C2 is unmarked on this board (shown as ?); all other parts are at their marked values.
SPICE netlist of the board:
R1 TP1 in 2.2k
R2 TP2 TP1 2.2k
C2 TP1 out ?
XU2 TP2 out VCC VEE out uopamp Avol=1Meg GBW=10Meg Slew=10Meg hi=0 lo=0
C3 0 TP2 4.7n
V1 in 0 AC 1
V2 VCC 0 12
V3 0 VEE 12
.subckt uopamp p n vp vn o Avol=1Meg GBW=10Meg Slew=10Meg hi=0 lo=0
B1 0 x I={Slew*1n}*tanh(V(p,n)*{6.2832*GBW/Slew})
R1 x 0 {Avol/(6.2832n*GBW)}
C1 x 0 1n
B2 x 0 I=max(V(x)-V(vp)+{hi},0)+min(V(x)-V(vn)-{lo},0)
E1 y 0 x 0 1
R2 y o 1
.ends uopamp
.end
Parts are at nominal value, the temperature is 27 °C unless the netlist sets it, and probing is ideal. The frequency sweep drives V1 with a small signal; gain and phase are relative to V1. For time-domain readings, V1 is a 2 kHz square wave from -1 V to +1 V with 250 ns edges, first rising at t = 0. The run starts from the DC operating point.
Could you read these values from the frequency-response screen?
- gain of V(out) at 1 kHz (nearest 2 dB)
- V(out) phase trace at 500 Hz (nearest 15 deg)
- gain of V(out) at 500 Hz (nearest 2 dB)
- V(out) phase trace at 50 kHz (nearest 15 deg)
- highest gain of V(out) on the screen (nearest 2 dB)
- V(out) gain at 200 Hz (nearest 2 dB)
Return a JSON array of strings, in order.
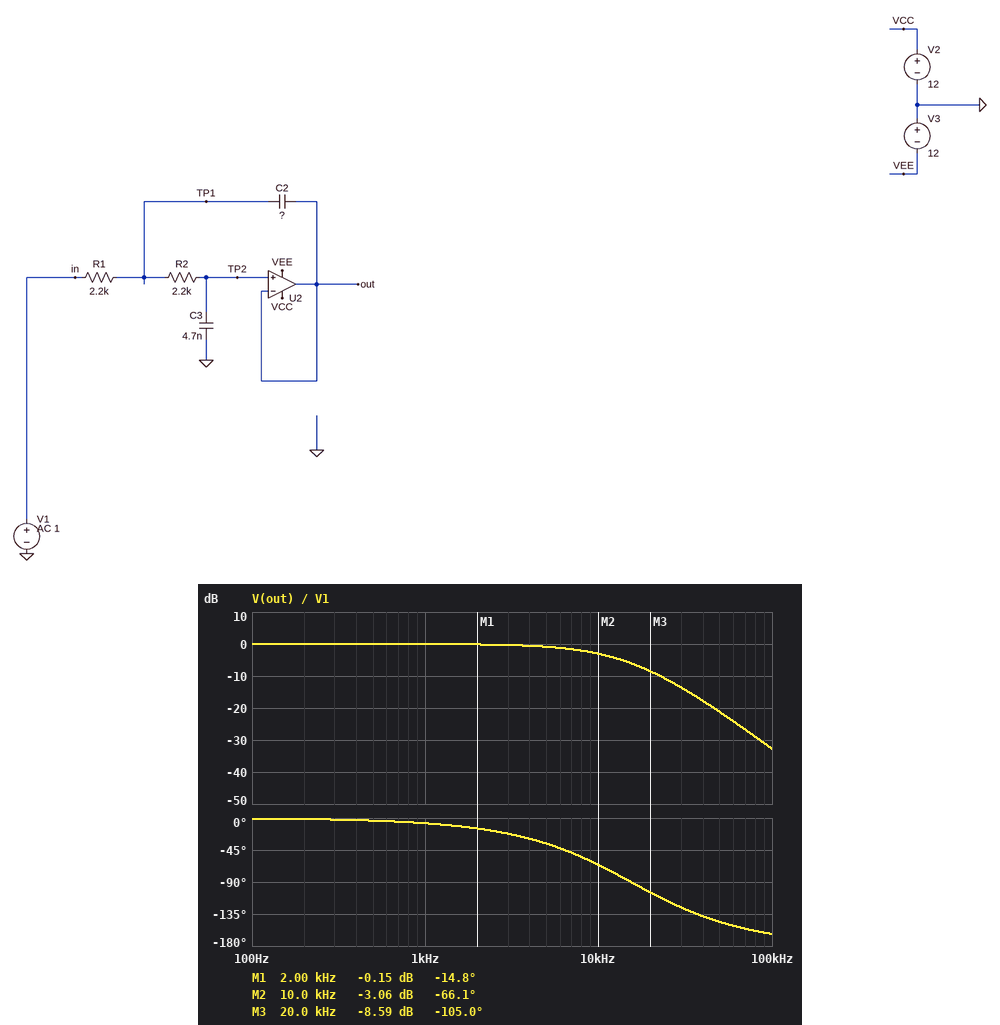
["0 dB", "0 deg", "0 dB", "-150 deg", "0 dB", "0 dB"]
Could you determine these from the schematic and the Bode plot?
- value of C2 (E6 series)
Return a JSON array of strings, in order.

["4.7 nF"]
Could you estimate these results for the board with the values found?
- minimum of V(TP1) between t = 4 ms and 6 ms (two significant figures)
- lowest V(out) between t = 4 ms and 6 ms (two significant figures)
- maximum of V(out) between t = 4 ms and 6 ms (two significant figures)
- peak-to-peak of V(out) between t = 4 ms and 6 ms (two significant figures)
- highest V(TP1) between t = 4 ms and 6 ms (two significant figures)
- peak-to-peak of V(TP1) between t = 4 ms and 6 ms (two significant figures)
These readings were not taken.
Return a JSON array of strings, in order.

["-1.0 V", "-1.0 V", "1.0 V", "2.0 V", "1.0 V", "2.0 V"]
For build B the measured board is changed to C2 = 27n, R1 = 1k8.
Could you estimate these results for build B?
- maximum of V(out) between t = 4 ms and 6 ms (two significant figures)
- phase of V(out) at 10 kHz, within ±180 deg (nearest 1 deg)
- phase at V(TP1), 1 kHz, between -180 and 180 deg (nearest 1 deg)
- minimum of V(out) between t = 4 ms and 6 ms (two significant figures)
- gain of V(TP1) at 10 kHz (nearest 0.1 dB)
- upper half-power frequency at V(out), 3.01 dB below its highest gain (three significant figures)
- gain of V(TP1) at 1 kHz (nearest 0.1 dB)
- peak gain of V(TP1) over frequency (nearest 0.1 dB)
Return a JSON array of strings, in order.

["1.5 V", "-130 deg", "-3 deg", "-1.5 V", "-2.2 dB", "8.42 kHz", "0.1 dB", "3.0 dB"]
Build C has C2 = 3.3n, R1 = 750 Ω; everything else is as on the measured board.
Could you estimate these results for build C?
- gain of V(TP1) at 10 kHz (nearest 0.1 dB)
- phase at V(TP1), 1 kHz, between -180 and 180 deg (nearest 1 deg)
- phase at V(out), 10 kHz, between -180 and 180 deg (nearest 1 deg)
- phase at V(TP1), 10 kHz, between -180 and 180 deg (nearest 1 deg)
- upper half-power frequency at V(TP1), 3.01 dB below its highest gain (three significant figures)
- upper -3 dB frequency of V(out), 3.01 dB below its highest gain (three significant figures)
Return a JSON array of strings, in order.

["-0.4 dB", "-1 deg", "-44 deg", "-11 deg", "55.9 kHz", "13.2 kHz"]
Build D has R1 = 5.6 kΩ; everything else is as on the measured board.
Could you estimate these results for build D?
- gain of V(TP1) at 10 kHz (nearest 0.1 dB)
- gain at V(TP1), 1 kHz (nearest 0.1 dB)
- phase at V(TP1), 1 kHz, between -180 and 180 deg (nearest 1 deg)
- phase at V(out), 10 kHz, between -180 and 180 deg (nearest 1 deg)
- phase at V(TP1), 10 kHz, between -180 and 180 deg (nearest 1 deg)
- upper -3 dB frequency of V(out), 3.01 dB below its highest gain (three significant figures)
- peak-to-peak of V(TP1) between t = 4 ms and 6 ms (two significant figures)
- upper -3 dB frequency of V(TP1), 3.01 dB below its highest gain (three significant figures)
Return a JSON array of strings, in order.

["-5.7 dB", "-0.1 dB", "-9 deg", "-92 deg", "-59 deg", "5.36 kHz", "2.0 V", "6.05 kHz"]
